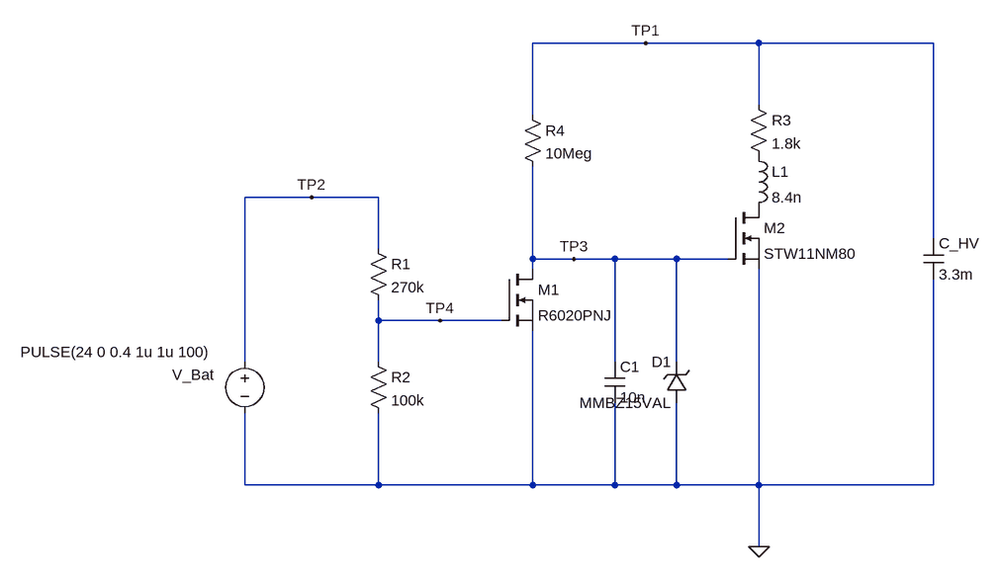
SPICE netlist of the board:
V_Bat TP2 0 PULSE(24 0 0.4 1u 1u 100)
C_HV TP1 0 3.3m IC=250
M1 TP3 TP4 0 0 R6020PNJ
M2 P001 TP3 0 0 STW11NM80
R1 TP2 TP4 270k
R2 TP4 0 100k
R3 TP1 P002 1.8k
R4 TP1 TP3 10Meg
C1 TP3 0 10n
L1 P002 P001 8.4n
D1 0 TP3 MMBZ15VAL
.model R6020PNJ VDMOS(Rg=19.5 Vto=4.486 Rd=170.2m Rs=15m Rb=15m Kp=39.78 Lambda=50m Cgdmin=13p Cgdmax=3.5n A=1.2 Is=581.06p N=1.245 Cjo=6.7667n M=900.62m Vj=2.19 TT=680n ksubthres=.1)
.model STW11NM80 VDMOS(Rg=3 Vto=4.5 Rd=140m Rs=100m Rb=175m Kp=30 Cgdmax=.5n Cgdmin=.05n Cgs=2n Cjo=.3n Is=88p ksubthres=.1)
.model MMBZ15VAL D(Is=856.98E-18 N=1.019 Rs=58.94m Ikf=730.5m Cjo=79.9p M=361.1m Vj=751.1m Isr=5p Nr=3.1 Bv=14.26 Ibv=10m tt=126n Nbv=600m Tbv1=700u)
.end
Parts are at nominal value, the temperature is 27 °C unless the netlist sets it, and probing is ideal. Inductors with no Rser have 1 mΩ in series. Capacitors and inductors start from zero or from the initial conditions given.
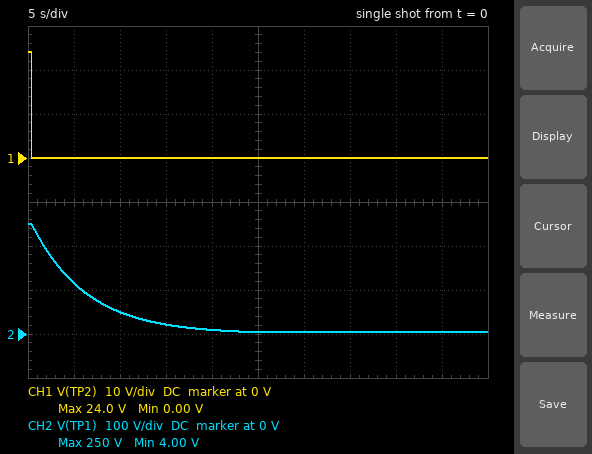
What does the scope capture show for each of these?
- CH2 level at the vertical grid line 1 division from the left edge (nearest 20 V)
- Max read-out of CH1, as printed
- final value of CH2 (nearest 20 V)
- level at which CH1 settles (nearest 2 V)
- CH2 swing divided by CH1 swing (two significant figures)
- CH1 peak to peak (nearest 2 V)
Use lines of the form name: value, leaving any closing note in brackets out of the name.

CH2 level at the vertical grid line 1 division from the left edge: 120 V
Max read-out of CH1, as printed: 24.0 V
final value of CH2: 0 V
level at which CH1 settles: 0 V
CH2 swing divided by CH1 swing: 10
CH1 peak to peak: 24 V
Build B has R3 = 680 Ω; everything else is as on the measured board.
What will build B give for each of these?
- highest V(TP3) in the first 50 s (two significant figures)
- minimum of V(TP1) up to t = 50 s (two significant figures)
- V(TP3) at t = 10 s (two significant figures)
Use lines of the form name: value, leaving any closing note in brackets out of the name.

highest V(TP3) in the first 50 s: 14 V
minimum of V(TP1) up to t = 50 s: 3.9 V
V(TP3) at t = 10 s: 4.0 V
